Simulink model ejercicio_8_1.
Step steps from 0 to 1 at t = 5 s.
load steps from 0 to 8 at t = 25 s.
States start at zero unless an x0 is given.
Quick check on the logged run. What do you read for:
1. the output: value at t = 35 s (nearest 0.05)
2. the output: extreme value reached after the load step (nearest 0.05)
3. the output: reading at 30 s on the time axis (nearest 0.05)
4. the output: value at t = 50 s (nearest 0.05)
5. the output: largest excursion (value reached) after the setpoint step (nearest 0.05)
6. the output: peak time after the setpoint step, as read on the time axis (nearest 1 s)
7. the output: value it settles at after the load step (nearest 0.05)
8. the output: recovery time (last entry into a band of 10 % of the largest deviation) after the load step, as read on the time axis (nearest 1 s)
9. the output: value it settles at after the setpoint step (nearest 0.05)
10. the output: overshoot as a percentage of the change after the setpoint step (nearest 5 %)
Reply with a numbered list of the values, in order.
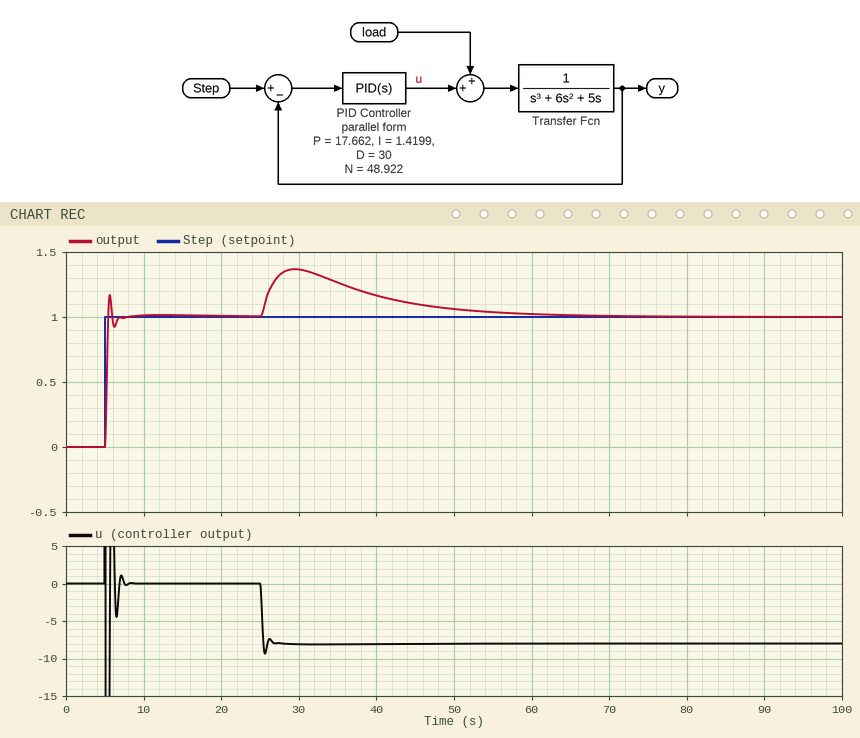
1. 1.25
2. 1.35
3. 1.35
4. 1.05
5. 1.15
6. 6 s
7. 1.00
8. 55 s
9. 1.00
10. 15 %
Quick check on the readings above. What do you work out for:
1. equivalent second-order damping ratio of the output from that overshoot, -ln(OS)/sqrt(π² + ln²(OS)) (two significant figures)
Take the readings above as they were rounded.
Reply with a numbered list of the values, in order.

1. 0.52
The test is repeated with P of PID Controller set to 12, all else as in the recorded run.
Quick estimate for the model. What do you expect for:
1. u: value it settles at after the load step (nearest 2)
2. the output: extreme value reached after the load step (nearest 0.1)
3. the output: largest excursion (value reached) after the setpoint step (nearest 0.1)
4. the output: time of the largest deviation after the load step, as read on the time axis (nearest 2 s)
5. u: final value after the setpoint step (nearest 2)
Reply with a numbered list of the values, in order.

1. -8
2. 1.5
3. 1.1
4. 30 s
5. 0
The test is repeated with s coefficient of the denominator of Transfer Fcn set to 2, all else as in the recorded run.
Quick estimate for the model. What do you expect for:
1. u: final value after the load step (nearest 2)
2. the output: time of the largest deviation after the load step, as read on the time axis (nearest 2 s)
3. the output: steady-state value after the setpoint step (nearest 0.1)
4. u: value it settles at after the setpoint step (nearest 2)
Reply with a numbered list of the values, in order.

1. -8
2. 30 s
3. 1.0
4. 0
